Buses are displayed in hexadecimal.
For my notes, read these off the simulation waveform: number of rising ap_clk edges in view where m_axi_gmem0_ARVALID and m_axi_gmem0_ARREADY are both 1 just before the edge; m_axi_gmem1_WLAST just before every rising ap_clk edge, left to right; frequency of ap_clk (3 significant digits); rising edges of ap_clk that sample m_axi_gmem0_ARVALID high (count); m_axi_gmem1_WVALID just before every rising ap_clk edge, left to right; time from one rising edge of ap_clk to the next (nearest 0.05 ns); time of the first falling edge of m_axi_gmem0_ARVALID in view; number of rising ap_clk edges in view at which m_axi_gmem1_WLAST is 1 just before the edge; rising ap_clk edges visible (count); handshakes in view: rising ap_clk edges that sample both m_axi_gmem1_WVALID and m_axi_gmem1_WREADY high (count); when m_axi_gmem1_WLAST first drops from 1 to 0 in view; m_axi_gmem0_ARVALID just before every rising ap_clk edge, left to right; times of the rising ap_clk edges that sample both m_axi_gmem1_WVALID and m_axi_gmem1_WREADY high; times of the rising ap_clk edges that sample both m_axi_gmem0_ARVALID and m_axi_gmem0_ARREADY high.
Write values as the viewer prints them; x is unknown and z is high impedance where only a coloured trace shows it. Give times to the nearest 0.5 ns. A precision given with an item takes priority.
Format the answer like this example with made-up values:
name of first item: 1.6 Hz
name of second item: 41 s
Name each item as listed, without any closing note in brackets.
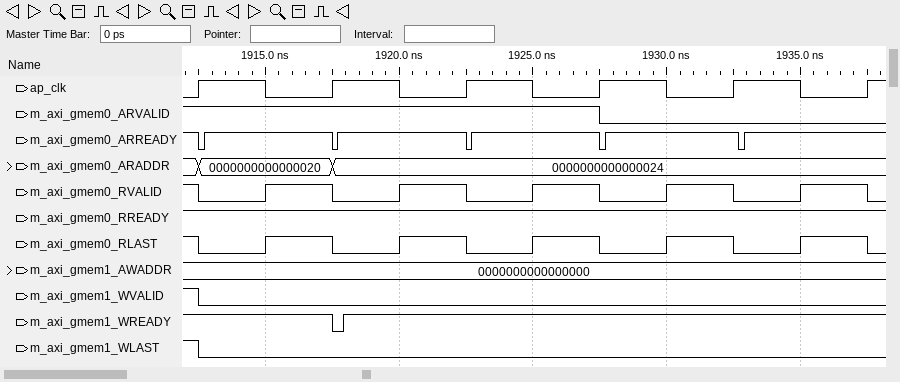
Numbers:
number of rising ap_clk edges in view where m_axi_gmem0_ARVALID and m_axi_gmem0_ARREADY are both 1 just before the edge: 4
m_axi_gmem1_WLAST just before every rising ap_clk edge, left to right: 1 0 0 0 0 0
frequency of ap_clk: 200 MHz
rising edges of ap_clk that sample m_axi_gmem0_ARVALID high: 4
m_axi_gmem1_WVALID just before every rising ap_clk edge, left to right: 1 0 0 0 0 0
time from one rising edge of ap_clk to the next: 5 ns
time of the first falling edge of m_axi_gmem0_ARVALID in view: 1927.5 ns
number of rising ap_clk edges in view at which m_axi_gmem1_WLAST is 1 just before the edge: 1
rising ap_clk edges visible: 6
handshakes in view: rising ap_clk edges that sample both m_axi_gmem1_WVALID and m_axi_gmem1_WREADY high: 1
when m_axi_gmem1_WLAST first drops from 1 to 0 in view: 1912.5 ns
m_axi_gmem0_ARVALID just before every rising ap_clk edge, left to right: 1 1 1 1 0 0
times of the rising ap_clk edges that sample both m_axi_gmem1_WVALID and m_axi_gmem1_WREADY high: 1912.5 ns
times of the rising ap_clk edges that sample both m_axi_gmem0_ARVALID and m_axi_gmem0_ARREADY high: 1912.5 ns, 1917.5 ns, 1922.5 ns, 1927.5 ns
